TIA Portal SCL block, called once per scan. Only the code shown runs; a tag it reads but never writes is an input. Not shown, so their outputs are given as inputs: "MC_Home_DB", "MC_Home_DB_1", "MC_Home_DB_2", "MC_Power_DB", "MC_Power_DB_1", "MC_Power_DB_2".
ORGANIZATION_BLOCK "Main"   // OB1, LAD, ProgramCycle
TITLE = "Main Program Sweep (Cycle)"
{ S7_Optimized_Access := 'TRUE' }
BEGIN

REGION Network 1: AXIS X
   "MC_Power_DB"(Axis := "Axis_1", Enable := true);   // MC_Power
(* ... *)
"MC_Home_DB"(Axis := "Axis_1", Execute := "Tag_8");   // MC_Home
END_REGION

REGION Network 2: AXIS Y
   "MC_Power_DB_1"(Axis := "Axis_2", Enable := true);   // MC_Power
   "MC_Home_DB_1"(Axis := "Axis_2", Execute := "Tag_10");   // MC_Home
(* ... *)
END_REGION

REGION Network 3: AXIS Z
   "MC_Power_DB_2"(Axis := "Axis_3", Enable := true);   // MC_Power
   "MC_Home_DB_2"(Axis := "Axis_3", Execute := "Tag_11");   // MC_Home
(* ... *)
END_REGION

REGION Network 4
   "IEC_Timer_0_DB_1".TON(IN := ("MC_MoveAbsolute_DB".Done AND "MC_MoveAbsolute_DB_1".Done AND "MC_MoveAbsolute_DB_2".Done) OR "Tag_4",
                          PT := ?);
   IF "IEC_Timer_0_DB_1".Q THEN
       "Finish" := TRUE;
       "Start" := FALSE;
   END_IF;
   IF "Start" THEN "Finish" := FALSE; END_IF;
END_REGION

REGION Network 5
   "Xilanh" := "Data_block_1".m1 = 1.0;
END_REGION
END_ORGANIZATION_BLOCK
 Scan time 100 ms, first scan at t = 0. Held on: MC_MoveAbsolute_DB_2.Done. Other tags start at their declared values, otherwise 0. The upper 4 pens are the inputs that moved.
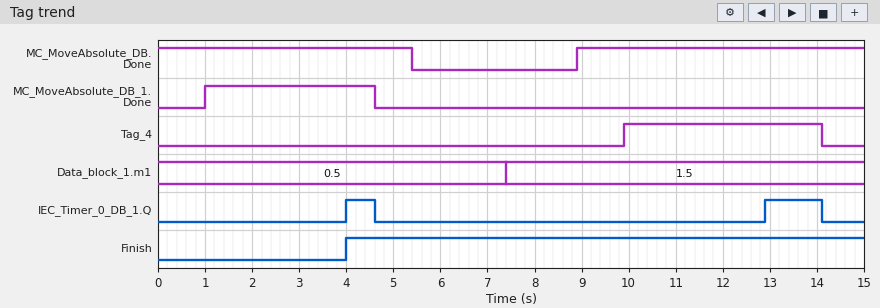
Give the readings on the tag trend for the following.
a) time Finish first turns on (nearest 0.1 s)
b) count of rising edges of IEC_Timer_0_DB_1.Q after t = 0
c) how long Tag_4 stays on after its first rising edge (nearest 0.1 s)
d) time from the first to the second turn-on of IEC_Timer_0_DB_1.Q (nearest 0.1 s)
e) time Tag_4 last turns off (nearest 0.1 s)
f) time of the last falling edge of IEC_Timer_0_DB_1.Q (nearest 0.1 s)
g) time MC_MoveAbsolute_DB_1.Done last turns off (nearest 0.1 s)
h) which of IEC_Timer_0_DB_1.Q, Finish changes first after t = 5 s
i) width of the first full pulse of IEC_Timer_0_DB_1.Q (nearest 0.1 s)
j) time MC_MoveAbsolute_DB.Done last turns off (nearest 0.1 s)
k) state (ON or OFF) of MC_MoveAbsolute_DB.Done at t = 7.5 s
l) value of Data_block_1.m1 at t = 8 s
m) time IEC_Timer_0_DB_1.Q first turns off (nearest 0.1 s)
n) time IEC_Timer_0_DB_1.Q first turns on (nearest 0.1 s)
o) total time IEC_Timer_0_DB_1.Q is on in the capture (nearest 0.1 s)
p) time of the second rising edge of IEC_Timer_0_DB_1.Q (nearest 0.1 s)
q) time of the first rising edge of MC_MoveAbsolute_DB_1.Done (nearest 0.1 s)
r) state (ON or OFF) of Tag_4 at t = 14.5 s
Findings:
4.0 s
2
4.2 s
8.9 s
14.1 s
14.1 s
4.6 s
IEC_Timer_0_DB_1.Q
0.6 s
5.4 s
OFF
1.5
4.6 s
4.0 s
1.8 s
12.9 s
1.0 s
OFF
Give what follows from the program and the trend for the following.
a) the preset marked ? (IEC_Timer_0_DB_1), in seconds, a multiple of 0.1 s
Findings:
3.0 s
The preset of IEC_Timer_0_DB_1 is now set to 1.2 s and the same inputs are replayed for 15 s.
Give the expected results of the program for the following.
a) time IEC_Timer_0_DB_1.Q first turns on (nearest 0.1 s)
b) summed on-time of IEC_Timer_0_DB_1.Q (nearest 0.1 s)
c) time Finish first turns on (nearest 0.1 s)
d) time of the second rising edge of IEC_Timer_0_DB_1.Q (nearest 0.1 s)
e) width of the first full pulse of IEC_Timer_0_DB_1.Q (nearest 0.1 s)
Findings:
2.2 s
5.4 s
2.2 s
11.1 s
2.4 s
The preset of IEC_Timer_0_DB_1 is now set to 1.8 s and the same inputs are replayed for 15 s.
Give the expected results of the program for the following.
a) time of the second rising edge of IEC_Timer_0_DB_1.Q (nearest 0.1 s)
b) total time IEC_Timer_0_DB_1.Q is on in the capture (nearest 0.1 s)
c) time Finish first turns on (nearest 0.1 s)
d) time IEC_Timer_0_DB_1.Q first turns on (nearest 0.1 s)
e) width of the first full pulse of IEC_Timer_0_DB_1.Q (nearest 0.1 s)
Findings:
11.7 s
4.2 s
2.8 s
2.8 s
1.8 s
